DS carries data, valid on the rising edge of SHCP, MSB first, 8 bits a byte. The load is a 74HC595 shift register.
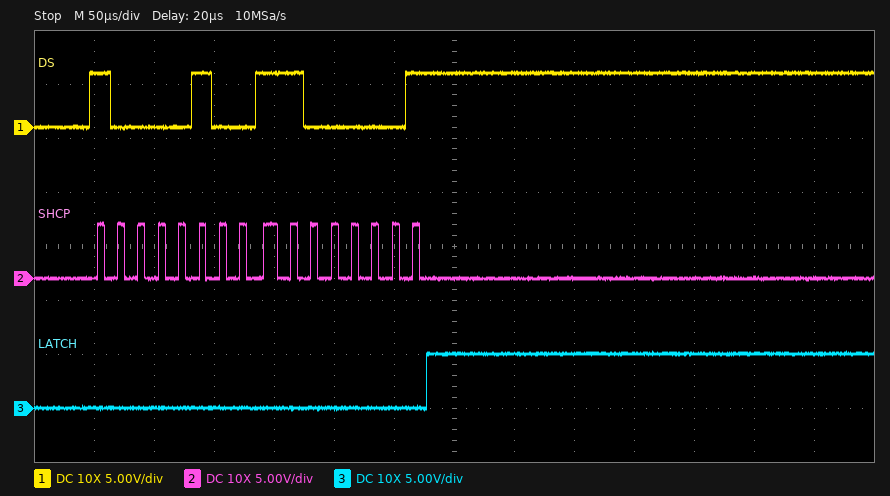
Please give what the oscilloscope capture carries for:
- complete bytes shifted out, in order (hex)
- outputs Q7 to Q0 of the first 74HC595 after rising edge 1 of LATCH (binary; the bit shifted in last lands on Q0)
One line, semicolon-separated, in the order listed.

0x84 0xC1; 11000001
